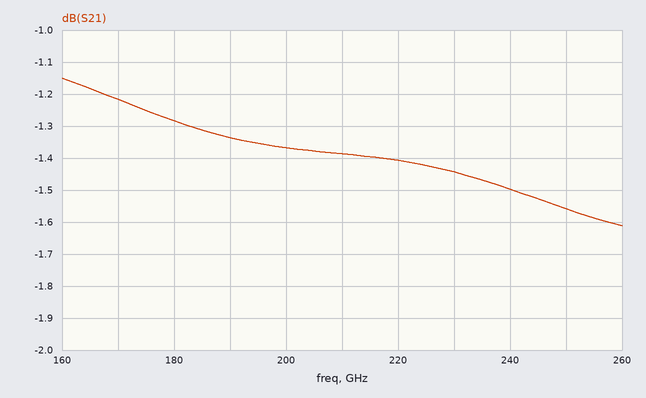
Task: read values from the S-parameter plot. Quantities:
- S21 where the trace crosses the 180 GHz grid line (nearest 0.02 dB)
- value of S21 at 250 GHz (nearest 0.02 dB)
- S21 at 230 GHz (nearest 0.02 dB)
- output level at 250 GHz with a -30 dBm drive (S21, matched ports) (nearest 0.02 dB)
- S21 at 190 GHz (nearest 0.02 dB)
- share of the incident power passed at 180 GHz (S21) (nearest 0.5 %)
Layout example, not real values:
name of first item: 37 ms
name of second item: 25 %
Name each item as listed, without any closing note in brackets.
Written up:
S21 where the trace crosses the 180 GHz grid line: -1.28 dB
value of S21 at 250 GHz: -1.56 dB
S21 at 230 GHz: -1.44 dB
output level at 250 GHz with a -30 dBm drive (S21, matched ports): -31.56 dBm
S21 at 190 GHz: -1.34 dB
share of the incident power passed at 180 GHz (S21): 74.5 %
